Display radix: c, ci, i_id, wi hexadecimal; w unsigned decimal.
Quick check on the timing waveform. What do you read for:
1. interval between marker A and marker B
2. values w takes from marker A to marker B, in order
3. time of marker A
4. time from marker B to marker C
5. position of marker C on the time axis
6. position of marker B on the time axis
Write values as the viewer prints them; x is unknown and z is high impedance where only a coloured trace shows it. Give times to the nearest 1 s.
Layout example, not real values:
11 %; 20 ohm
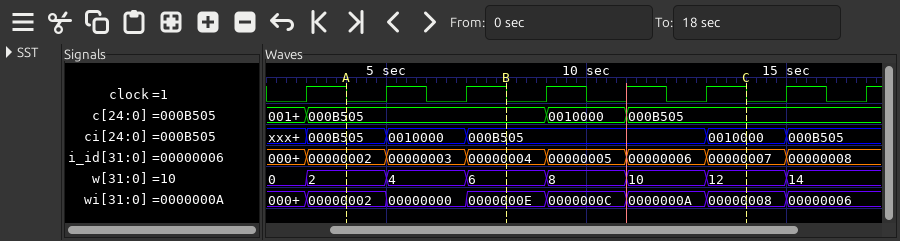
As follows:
4 s; 2, 4, 6; 4 s; 6 s; 14 s; 8 s
